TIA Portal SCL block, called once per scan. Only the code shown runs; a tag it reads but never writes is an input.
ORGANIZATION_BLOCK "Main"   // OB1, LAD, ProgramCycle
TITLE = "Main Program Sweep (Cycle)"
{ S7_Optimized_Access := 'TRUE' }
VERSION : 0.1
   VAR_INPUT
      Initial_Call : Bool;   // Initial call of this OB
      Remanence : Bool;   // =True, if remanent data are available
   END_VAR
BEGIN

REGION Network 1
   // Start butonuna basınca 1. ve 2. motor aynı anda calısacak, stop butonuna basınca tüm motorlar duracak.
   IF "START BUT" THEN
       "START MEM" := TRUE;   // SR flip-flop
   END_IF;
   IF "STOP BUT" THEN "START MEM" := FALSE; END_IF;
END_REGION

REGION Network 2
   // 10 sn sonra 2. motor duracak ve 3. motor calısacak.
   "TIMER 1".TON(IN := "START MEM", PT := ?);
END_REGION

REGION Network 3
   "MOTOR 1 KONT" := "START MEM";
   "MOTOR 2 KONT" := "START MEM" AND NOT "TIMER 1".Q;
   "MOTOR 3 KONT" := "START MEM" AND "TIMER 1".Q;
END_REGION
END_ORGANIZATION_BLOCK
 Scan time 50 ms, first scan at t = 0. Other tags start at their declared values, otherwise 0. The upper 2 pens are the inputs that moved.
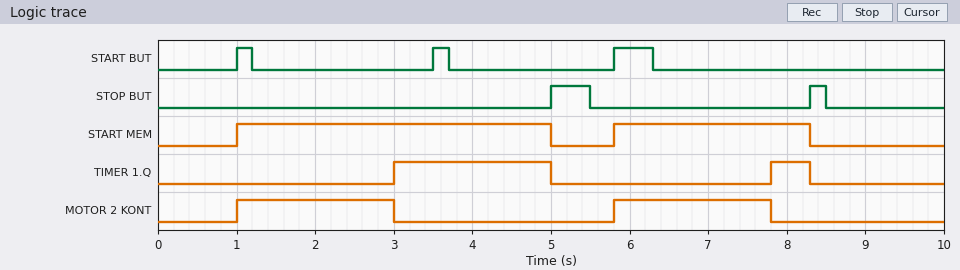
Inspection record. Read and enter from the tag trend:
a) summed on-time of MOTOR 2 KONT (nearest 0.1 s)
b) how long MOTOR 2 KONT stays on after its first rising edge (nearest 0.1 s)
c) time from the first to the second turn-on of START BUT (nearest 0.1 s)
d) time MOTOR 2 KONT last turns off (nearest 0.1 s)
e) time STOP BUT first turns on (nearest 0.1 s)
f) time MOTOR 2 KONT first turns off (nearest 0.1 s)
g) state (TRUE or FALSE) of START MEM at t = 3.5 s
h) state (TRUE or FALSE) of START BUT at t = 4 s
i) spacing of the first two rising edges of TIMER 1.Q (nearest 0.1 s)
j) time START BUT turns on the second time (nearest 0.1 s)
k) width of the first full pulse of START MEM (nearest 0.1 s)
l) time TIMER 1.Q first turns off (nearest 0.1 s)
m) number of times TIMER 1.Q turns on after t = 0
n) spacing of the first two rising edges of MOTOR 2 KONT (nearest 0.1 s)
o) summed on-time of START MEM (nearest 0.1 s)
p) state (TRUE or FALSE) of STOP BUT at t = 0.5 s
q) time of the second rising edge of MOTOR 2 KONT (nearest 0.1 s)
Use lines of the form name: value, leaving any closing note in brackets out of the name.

summed on-time of MOTOR 2 KONT: 4.0 s
how long MOTOR 2 KONT stays on after its first rising edge: 2.0 s
time from the first to the second turn-on of START BUT: 2.5 s
time MOTOR 2 KONT last turns off: 7.8 s
time STOP BUT first turns on: 5.0 s
time MOTOR 2 KONT first turns off: 3.0 s
state (TRUE or FALSE) of START MEM at t = 3.5 s: TRUE
state (TRUE or FALSE) of START BUT at t = 4 s: FALSE
spacing of the first two rising edges of TIMER 1.Q: 4.8 s
time START BUT turns on the second time: 3.5 s
width of the first full pulse of START MEM: 4.0 s
time TIMER 1.Q first turns off: 5.0 s
number of times TIMER 1.Q turns on after t = 0: 2
spacing of the first two rising edges of MOTOR 2 KONT: 4.8 s
summed on-time of START MEM: 6.5 s
state (TRUE or FALSE) of STOP BUT at t = 0.5 s: FALSE
time of the second rising edge of MOTOR 2 KONT: 5.8 s
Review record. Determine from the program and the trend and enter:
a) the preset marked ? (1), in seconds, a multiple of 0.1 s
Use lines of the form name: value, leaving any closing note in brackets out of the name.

the preset marked ? (1), in seconds, a multiple of 0.1 s: 2.0 s
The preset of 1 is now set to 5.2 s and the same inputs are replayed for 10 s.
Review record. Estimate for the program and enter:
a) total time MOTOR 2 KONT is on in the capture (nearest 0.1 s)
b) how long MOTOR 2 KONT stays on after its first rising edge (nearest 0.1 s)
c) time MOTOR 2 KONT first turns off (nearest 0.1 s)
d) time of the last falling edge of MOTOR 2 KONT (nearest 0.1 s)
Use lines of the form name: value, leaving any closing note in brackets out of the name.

total time MOTOR 2 KONT is on in the capture: 6.5 s
how long MOTOR 2 KONT stays on after its first rising edge: 4.0 s
time MOTOR 2 KONT first turns off: 5.0 s
time of the last falling edge of MOTOR 2 KONT: 8.3 s
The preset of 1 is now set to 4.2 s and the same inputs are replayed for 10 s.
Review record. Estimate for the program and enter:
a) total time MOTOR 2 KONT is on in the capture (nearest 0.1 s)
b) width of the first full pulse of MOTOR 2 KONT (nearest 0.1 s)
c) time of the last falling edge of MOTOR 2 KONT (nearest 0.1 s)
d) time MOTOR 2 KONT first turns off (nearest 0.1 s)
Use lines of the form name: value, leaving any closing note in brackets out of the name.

total time MOTOR 2 KONT is on in the capture: 6.5 s
width of the first full pulse of MOTOR 2 KONT: 4.0 s
time of the last falling edge of MOTOR 2 KONT: 8.3 s
time MOTOR 2 KONT first turns off: 5.0 s
